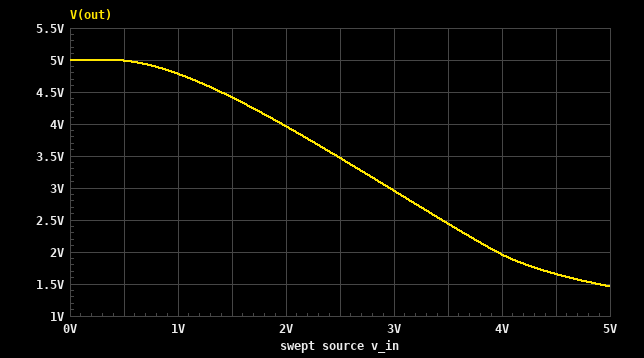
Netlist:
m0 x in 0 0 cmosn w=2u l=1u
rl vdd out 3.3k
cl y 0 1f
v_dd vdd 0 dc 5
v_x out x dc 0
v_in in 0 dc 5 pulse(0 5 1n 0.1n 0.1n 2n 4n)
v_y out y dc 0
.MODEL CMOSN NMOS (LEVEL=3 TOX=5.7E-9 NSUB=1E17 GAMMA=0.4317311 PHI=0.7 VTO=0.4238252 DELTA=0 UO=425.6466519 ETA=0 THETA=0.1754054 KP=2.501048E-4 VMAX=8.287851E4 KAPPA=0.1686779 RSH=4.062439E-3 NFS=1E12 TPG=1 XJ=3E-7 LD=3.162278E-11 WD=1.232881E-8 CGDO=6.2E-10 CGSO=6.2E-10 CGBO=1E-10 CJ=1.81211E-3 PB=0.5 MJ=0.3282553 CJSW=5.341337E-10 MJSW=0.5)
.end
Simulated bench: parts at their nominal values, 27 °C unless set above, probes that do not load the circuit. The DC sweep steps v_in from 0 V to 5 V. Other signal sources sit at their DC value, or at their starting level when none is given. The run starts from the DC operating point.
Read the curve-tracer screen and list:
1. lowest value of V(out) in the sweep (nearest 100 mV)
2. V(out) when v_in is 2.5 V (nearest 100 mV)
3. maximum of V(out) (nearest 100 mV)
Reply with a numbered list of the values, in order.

1. 1.5 V
2. 3.5 V
3. 5.0 V
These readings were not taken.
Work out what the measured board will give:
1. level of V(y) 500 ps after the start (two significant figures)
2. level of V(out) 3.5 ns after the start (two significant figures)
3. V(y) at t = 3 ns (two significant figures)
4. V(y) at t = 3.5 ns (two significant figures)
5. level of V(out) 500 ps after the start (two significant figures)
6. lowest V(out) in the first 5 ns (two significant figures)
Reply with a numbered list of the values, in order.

1. 5.0 V
2. 5.0 V
3. 1.5 V
4. 5.0 V
5. 5.0 V
6. 1.3 V
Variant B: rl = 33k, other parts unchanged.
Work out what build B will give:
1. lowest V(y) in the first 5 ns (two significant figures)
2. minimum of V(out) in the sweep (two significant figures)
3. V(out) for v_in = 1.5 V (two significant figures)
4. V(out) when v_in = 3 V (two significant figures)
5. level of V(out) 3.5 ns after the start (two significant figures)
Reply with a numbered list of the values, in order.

1. -620 mV
2. 120 mV
3. 470 mV
4. 180 mV
5. 4.9 V
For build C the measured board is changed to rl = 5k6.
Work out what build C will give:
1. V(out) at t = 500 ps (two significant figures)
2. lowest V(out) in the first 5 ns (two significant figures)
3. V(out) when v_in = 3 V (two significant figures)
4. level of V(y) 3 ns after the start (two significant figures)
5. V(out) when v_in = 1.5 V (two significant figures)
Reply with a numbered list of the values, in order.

1. 5.0 V
2. 540 mV
3. 1.7 V
4. 810 mV
5. 4.0 V
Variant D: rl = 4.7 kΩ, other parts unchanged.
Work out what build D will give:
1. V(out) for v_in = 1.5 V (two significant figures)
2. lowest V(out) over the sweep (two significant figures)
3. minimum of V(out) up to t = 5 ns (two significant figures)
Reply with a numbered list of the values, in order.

1. 4.2 V
2. 990 mV
3. 730 mV
